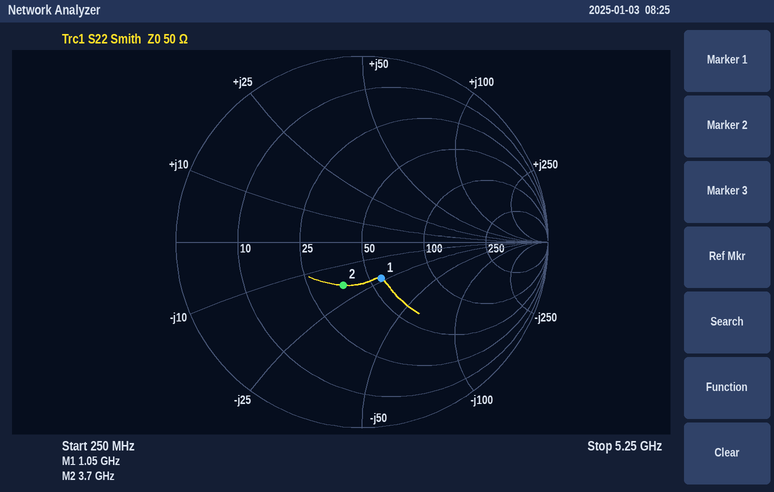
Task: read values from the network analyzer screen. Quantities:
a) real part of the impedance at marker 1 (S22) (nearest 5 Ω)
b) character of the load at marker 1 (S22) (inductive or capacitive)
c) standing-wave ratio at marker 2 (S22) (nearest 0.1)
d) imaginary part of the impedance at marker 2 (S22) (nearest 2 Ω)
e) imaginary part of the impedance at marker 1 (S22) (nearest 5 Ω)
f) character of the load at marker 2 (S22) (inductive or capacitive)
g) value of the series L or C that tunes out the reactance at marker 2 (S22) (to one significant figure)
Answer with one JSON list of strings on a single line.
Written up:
["55 Ω", "capacitive", "1.7", "-18 Ω", "-25 Ω", "capacitive", "800 pH"]
